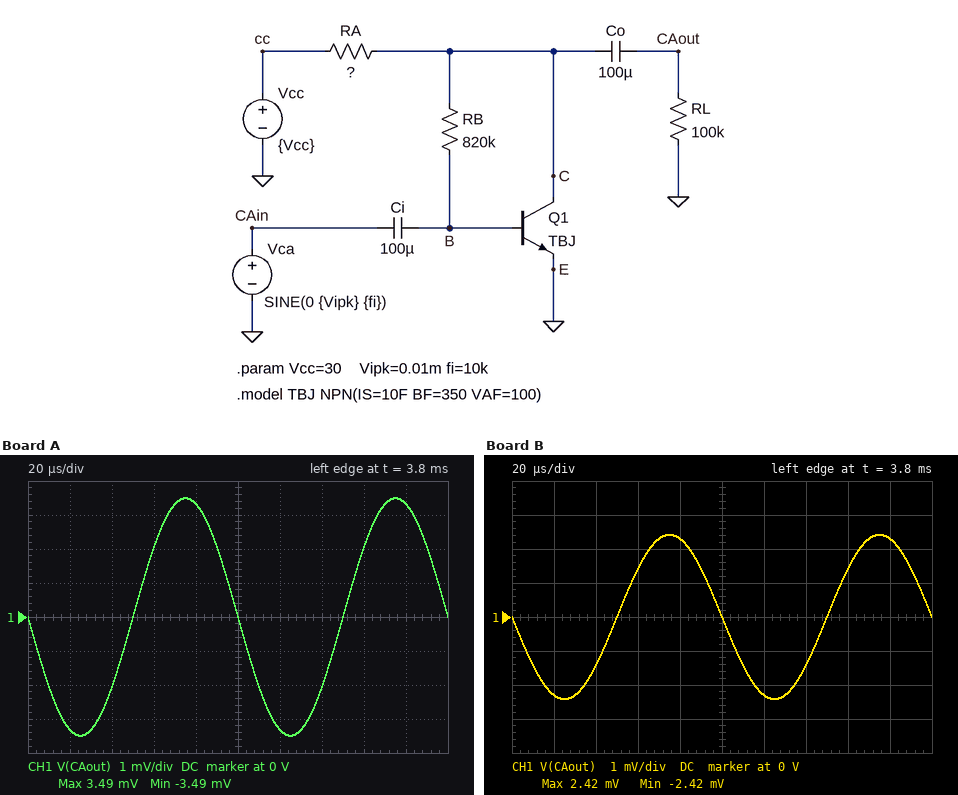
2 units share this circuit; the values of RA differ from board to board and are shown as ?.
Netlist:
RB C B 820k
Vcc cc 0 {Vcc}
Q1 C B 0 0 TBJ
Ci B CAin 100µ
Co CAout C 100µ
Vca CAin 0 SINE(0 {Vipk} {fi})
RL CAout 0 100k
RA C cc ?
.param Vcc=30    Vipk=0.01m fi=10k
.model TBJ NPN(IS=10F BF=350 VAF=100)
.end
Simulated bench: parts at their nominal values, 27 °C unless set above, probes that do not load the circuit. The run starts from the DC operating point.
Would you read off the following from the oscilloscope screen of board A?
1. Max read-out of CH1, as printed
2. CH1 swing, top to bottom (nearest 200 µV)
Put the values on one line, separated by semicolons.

3.49 mV; 7.0 mV
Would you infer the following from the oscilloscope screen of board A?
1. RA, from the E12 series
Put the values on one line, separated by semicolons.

1 kΩ
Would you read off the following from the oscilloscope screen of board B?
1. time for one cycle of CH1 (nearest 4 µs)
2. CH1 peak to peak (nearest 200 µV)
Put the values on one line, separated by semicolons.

100 µs; 4.8 mV
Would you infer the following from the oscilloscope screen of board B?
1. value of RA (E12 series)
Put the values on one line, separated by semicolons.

560 Ω
